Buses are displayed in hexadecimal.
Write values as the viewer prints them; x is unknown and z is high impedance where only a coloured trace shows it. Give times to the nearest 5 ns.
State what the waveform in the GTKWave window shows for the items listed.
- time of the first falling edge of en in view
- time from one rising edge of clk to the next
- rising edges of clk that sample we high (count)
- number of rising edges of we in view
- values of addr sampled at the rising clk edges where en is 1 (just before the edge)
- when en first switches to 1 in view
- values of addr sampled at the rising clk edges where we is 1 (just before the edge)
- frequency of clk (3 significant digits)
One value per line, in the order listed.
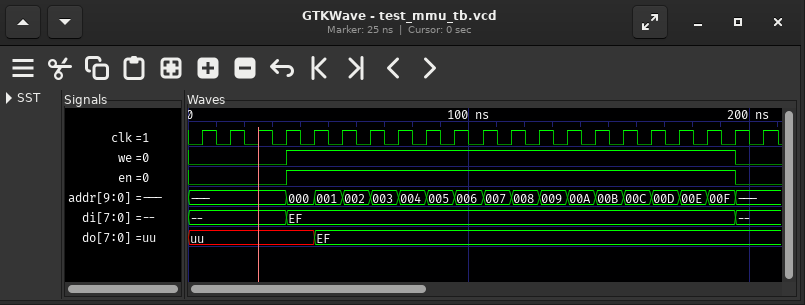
195 ns
10 ns
16
1
000, 001, 002, 003, 004, 005, 006, 007, 008, 009, 00A, 00B, 00C, 00D, 00E, 00F
35 ns
000, 001, 002, 003, 004, 005, 006, 007, 008, 009, 00A, 00B, 00C, 00D, 00E, 00F
100 MHz
